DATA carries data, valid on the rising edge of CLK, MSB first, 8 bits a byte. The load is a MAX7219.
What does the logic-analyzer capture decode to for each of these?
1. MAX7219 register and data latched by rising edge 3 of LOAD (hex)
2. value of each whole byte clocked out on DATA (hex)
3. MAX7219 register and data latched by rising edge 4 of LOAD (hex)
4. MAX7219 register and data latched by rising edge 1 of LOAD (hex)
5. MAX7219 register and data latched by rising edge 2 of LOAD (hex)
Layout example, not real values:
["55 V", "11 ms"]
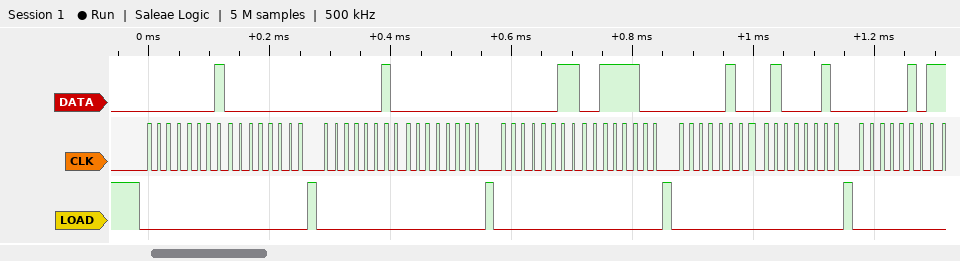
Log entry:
["register 0x3, data 0x3C", "01 00 02 00 03 3C 04 42 05", "register 0x4, data 0x42", "register 0x1, data 0x00", "register 0x2, data 0x00"]
